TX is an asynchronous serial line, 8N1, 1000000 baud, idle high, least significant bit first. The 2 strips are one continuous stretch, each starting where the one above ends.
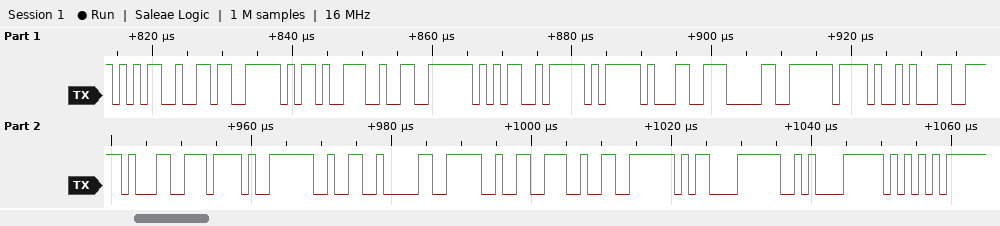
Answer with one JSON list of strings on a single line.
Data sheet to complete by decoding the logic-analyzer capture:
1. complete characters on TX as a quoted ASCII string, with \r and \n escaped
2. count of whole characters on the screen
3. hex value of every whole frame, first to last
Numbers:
["\"56-25_10/11/2022\\r\\nU\"", "19", "35 36 2D 32 35 5F 31 30 2F 31 31 2F 32 30 32 32 0D 0A 55"]
